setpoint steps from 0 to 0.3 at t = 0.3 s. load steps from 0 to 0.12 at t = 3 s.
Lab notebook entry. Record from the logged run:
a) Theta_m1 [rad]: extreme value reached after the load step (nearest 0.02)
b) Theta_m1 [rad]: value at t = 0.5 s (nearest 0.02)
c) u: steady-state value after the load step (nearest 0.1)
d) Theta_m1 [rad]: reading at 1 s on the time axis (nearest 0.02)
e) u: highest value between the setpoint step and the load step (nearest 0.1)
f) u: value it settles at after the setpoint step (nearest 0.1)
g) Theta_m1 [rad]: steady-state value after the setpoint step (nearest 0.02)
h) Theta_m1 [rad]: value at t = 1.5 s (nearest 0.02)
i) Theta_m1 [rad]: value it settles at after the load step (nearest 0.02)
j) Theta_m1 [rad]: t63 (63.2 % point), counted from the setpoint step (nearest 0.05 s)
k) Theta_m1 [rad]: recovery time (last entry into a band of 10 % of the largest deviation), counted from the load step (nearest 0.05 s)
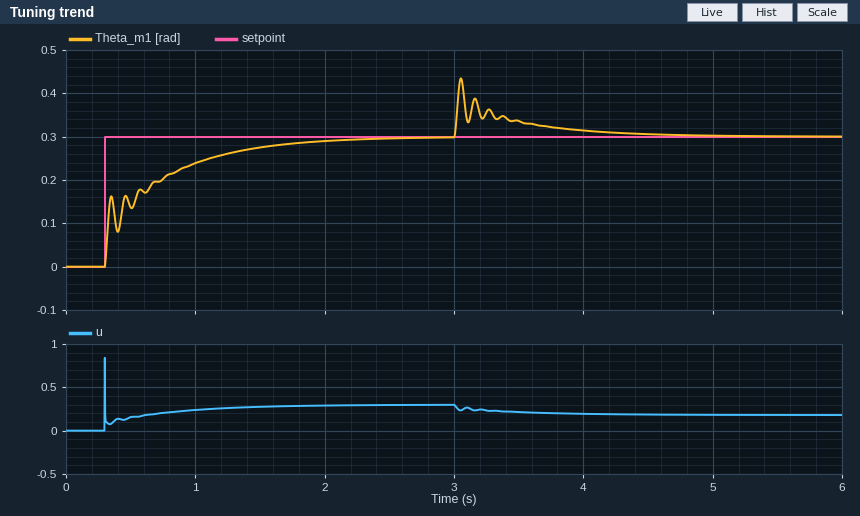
0.44
0.14
0.2
0.24
0.8
0.3
0.30
0.28
0.30
0.35 s
1.00 s
